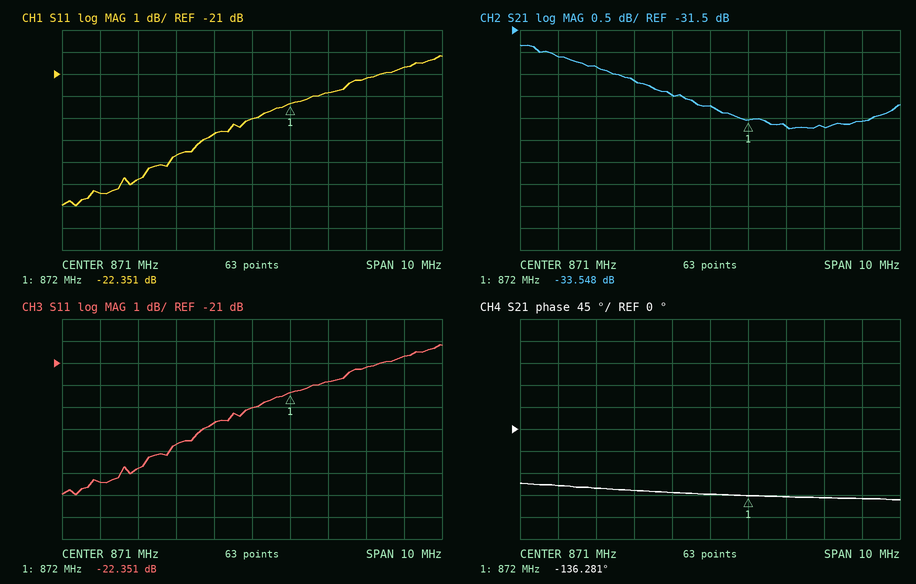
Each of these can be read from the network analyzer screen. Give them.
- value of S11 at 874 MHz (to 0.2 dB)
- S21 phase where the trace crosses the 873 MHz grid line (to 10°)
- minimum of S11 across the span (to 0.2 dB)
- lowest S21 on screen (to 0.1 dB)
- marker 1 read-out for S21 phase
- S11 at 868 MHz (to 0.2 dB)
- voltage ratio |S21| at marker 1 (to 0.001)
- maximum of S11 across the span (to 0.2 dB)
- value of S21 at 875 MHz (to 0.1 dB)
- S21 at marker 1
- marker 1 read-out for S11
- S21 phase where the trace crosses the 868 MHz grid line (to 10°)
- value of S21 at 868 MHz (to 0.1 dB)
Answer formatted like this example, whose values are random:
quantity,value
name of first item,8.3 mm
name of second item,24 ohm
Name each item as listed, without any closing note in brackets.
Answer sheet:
quantity,value
value of S11 at 874 MHz,-21.2 dB
S21 phase where the trace crosses the 873 MHz grid line,-140°
minimum of S11 across the span,-27.0 dB
lowest S21 on screen,-33.7 dB
marker 1 read-out for S21 phase,-136.281°
S11 at 868 MHz,-25.8 dB
voltage ratio |S21| at marker 1,0.021
maximum of S11 across the span,-20.2 dB
value of S21 at 875 MHz,-33.6 dB
S21 at marker 1,-33.548 dB
marker 1 read-out for S11,-22.351 dB
S21 phase where the trace crosses the 868 MHz grid line,-120°
value of S21 at 868 MHz,-32.3 dB
